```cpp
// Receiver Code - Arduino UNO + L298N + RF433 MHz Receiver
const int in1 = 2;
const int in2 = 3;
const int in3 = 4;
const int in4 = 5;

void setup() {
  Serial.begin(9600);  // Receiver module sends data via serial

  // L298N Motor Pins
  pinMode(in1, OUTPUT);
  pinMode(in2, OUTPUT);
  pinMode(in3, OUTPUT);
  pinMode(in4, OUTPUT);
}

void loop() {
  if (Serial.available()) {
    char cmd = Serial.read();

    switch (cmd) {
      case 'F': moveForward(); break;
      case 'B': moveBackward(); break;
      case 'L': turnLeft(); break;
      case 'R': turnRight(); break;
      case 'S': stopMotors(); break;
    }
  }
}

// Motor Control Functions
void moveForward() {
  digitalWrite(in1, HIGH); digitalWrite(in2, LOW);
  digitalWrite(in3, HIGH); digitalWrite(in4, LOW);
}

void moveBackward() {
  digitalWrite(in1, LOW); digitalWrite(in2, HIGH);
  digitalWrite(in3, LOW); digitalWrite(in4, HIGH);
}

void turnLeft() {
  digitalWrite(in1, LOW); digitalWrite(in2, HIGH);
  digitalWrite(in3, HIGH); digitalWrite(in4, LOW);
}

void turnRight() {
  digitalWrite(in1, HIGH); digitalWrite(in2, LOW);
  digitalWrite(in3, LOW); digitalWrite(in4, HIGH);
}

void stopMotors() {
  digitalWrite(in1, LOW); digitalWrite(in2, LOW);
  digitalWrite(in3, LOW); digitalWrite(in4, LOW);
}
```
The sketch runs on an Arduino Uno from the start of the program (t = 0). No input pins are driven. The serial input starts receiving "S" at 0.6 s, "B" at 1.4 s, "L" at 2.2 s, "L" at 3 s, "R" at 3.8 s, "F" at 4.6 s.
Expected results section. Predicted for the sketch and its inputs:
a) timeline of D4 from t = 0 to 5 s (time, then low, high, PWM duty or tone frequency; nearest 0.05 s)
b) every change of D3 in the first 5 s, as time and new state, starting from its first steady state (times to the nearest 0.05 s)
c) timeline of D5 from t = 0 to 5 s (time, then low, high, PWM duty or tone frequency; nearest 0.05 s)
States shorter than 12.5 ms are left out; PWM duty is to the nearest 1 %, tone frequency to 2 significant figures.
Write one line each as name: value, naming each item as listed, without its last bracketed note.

timeline of D4 from t = 0 to 5 s: 0 s low; 2.2 s high; 3.8 s low; 4.6 s high
every change of D3 in the first 5 s, as time and new state, starting from its first steady state: 0 s low; 1.4 s high; 3.8 s low
timeline of D5 from t = 0 to 5 s: 0 s low; 1.4 s high; 2.2 s low; 3.8 s high; 4.6 s low
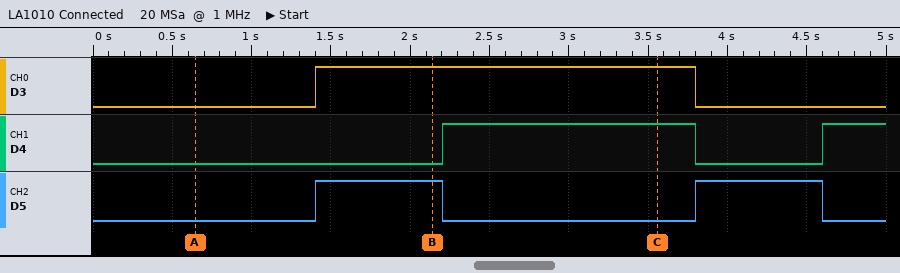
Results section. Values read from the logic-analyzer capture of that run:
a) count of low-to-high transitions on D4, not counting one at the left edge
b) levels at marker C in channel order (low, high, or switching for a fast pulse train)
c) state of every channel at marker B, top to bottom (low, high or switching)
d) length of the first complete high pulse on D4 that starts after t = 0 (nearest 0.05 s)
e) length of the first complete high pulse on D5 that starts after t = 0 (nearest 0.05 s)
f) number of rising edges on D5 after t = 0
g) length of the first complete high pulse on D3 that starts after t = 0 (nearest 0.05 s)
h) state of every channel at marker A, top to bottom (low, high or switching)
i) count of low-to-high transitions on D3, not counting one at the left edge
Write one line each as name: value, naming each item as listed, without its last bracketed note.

count of low-to-high transitions on D4, not counting one at the left edge: 2
levels at marker C in channel order: D3 high, D4 high, D5 low
state of every channel at marker B, top to bottom: D3 high, D4 low, D5 high
length of the first complete high pulse on D4 that starts after t = 0: 1.60 s
length of the first complete high pulse on D5 that starts after t = 0: 0.80 s
number of rising edges on D5 after t = 0: 2
length of the first complete high pulse on D3 that starts after t = 0: 2.40 s
state of every channel at marker A, top to bottom: D3 low, D4 low, D5 low
count of low-to-high transitions on D3, not counting one at the left edge: 1
